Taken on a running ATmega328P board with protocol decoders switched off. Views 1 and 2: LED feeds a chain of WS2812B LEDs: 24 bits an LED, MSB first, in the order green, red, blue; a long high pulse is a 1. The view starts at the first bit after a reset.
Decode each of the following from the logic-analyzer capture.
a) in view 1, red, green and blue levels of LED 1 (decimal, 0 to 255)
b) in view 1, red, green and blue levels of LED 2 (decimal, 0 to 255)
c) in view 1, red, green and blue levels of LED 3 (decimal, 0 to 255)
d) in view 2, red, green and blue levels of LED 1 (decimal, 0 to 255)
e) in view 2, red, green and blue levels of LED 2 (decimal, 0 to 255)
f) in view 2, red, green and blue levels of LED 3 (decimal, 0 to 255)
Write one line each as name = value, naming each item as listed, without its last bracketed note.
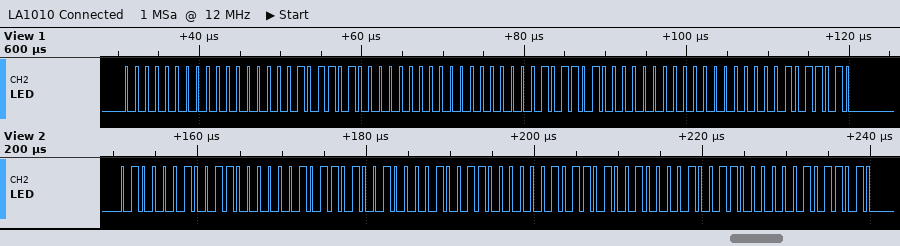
in view 1, red, green and blue levels of LED 1 = 0, 0, 90
in view 1, red, green and blue levels of LED 2 = 0, 0, 90
in view 1, red, green and blue levels of LED 3 = 0, 0, 90
in view 2, red, green and blue levels of LED 1 = 96, 66, 90
in view 2, red, green and blue levels of LED 2 = 96, 66, 90
in view 2, red, green and blue levels of LED 3 = 96, 66, 90
